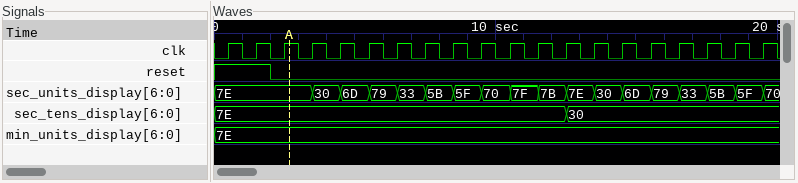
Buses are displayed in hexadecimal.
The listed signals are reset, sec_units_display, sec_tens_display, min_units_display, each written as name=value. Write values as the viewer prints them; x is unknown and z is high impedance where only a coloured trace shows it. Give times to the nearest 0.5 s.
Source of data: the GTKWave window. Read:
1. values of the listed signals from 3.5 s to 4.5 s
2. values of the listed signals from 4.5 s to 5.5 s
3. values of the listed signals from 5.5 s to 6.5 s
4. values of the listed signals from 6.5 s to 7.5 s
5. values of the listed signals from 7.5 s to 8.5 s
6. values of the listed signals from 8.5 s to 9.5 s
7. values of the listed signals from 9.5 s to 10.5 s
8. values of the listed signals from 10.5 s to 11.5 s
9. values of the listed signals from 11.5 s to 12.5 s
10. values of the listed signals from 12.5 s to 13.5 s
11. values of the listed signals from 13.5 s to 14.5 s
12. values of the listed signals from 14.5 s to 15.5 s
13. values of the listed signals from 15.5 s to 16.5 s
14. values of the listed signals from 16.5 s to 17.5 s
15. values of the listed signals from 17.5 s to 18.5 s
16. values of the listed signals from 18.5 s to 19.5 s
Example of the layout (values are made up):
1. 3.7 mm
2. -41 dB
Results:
1. reset=0, sec_units_display=30, sec_tens_display=7E, min_units_display=7E
2. reset=0, sec_units_display=6D, sec_tens_display=7E, min_units_display=7E
3. reset=0, sec_units_display=79, sec_tens_display=7E, min_units_display=7E
4. reset=0, sec_units_display=33, sec_tens_display=7E, min_units_display=7E
5. reset=0, sec_units_display=5B, sec_tens_display=7E, min_units_display=7E
6. reset=0, sec_units_display=5F, sec_tens_display=7E, min_units_display=7E
7. reset=0, sec_units_display=70, sec_tens_display=7E, min_units_display=7E
8. reset=0, sec_units_display=7F, sec_tens_display=7E, min_units_display=7E
9. reset=0, sec_units_display=7B, sec_tens_display=7E, min_units_display=7E
10. reset=0, sec_units_display=7E, sec_tens_display=30, min_units_display=7E
11. reset=0, sec_units_display=30, sec_tens_display=30, min_units_display=7E
12. reset=0, sec_units_display=6D, sec_tens_display=30, min_units_display=7E
13. reset=0, sec_units_display=79, sec_tens_display=30, min_units_display=7E
14. reset=0, sec_units_display=33, sec_tens_display=30, min_units_display=7E
15. reset=0, sec_units_display=5B, sec_tens_display=30, min_units_display=7E
16. reset=0, sec_units_display=5F, sec_tens_display=30, min_units_display=7E
